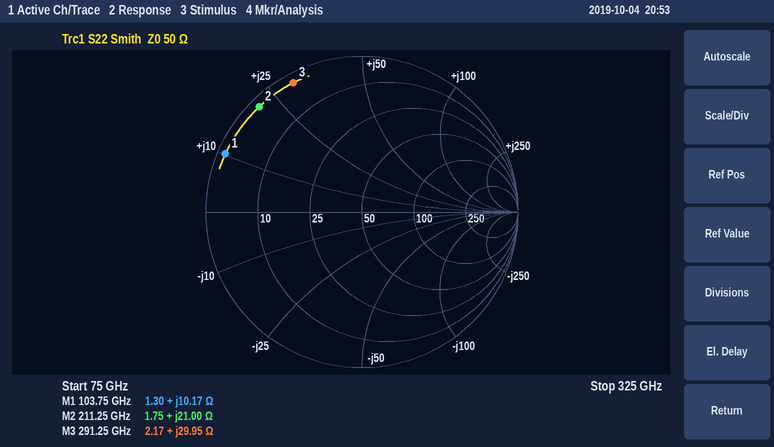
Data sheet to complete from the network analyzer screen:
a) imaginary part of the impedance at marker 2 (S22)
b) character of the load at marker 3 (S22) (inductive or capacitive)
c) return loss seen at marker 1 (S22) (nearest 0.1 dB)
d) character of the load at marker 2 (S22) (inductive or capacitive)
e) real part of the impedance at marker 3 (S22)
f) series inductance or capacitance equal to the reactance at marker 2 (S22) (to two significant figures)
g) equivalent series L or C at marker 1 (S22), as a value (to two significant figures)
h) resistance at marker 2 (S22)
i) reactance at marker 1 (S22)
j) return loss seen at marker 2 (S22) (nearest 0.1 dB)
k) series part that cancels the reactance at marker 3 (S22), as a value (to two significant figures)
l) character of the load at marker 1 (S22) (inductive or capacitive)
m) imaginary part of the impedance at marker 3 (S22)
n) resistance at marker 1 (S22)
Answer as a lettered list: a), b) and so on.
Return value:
a) +21.00 Ω
b) inductive
c) 0.4 dB
d) inductive
e) 2.17 Ω
f) 16 pH
g) 16 pH
h) 1.75 Ω
i) +10.17 Ω
j) 0.5 dB
k) 18 fF
l) inductive
m) +29.95 Ω
n) 1.30 Ω
